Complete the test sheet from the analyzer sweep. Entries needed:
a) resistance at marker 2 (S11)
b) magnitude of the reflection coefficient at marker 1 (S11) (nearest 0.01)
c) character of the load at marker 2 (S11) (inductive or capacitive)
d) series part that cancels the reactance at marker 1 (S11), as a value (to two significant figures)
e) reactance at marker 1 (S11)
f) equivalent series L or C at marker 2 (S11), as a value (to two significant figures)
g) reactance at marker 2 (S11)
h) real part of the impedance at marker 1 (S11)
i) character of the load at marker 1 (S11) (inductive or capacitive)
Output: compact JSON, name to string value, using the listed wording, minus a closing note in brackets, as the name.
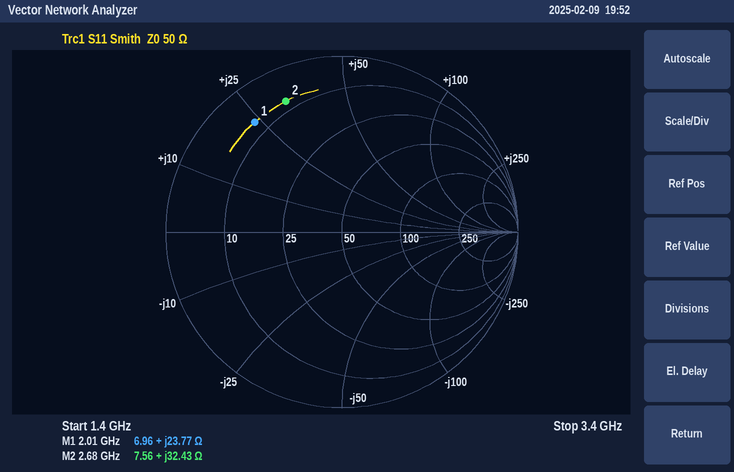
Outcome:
{"resistance at marker 2": "7.56 Ω", "magnitude of the reflection coefficient at marker 1 (S11)": "0.80", "character of the load at marker 2 (S11)": "inductive", "series part that cancels the reactance at marker 1 (S11), as a value": "3.3 pF", "reactance at marker 1": "+23.77 Ω", "equivalent series L or C at marker 2 (S11), as a value": "1.9 nH", "reactance at marker 2": "+32.43 Ω", "real part of the impedance at marker 1": "6.96 Ω", "character of the load at marker 1 (S11)": "inductive"}
